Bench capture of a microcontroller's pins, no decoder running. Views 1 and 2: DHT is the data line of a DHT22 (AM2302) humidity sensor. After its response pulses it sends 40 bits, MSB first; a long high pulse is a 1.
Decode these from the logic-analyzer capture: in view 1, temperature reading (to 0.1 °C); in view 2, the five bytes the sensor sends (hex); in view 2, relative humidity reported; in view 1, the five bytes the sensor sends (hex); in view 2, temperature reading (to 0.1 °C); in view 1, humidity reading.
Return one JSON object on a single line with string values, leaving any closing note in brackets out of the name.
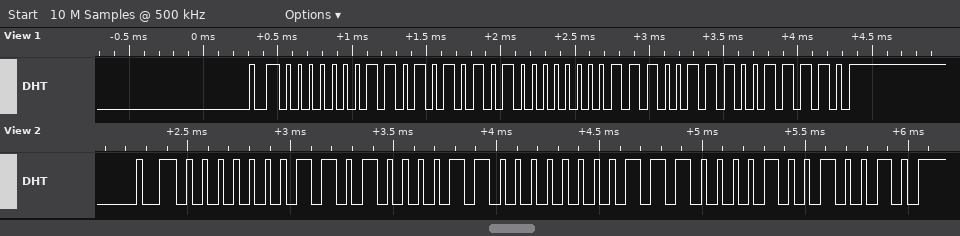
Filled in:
{"in view 1, temperature reading": "-11.5 °C", "in view 2, the five bytes the sensor sends": "01 A1 80 70 92", "in view 2, relative humidity reported": "41.7 %", "in view 1, the five bytes the sensor sends": "01 AA 80 73 9E", "in view 2, temperature reading": "-11.2 °C", "in view 1, humidity reading": "42.6 %"}
